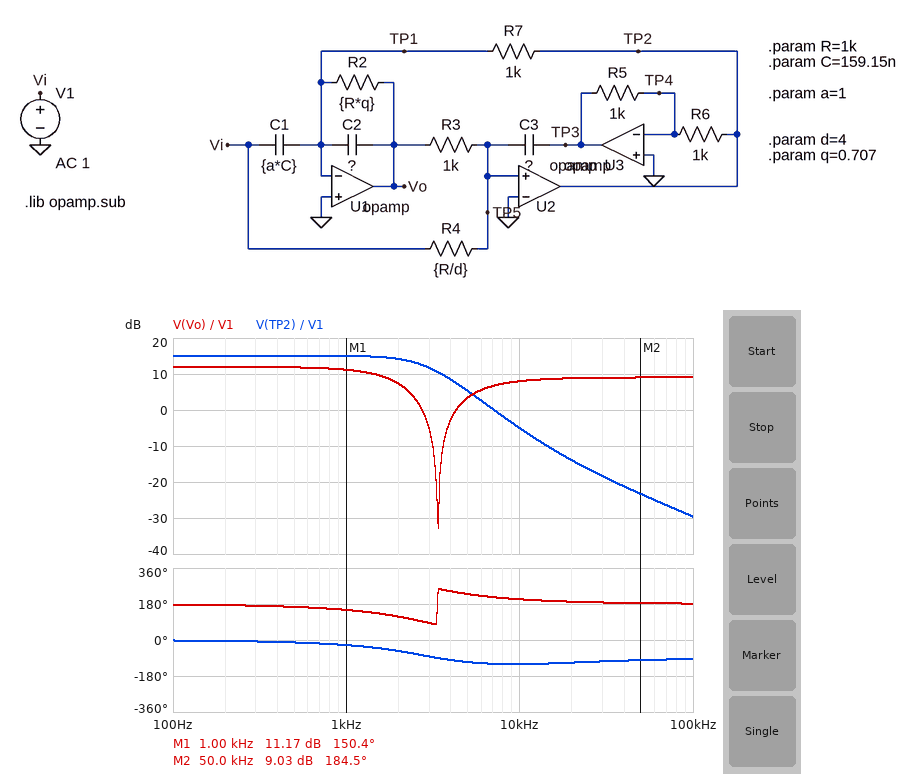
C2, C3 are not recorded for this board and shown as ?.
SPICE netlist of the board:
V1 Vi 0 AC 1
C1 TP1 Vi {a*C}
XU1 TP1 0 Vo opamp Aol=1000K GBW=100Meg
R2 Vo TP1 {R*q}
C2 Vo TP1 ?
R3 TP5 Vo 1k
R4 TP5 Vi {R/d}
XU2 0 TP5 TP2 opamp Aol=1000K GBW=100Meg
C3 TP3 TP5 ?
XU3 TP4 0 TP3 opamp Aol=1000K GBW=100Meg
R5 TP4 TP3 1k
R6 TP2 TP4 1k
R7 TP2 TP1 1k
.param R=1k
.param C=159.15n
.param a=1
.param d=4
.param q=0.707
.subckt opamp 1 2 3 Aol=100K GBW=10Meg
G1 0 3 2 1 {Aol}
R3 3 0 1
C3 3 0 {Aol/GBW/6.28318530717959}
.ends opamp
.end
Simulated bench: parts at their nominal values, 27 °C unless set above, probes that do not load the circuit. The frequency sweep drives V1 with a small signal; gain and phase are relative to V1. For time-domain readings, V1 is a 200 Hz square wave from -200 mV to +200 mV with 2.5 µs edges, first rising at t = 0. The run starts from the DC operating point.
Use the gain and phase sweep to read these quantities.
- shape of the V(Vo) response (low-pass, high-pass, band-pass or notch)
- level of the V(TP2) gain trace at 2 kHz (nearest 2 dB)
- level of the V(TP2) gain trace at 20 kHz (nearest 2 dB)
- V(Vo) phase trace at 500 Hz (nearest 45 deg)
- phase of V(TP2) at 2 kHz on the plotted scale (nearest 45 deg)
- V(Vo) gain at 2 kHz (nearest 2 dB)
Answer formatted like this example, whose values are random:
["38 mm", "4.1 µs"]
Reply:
["notch", "14 dB", "-14 dB", "180 deg", "-45 deg", "8 dB"]
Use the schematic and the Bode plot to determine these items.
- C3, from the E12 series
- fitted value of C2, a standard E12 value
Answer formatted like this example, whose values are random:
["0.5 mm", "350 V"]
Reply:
["56 nF", "56 nF"]
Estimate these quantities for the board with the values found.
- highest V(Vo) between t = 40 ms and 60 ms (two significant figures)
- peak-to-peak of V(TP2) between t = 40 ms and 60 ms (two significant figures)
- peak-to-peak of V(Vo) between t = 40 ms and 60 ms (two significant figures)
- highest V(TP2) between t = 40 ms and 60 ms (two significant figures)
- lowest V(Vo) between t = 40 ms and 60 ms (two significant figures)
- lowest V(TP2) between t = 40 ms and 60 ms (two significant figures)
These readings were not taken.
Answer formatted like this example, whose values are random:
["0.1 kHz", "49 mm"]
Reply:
["850 mV", "2.5 V", "1.7 V", "1.2 V", "-850 mV", "-1.2 V"]
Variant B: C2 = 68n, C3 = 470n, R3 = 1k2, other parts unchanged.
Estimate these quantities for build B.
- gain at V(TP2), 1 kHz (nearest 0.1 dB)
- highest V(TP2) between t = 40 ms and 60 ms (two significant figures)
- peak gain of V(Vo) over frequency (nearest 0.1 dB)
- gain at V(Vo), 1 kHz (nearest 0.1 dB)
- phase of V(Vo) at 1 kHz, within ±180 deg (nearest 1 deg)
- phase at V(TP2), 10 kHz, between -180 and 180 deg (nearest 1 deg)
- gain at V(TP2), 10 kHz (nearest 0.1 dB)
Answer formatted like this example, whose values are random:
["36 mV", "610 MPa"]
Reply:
["2.7 dB", "1.3 V", "13.6 dB", "-12.1 dB", "84 deg", "-104 deg", "-22.1 dB"]
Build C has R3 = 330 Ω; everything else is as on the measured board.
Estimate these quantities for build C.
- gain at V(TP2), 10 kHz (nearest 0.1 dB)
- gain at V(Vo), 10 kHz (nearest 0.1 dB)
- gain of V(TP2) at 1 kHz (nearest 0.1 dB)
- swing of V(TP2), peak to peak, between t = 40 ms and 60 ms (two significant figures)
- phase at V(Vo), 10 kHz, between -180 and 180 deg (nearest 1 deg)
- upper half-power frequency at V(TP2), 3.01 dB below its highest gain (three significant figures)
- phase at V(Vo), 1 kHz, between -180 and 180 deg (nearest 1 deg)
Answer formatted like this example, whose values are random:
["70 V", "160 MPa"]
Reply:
["4.2 dB", "9.4 dB", "6.0 dB", "1.5 V", "-152 deg", "6.83 kHz", "170 deg"]
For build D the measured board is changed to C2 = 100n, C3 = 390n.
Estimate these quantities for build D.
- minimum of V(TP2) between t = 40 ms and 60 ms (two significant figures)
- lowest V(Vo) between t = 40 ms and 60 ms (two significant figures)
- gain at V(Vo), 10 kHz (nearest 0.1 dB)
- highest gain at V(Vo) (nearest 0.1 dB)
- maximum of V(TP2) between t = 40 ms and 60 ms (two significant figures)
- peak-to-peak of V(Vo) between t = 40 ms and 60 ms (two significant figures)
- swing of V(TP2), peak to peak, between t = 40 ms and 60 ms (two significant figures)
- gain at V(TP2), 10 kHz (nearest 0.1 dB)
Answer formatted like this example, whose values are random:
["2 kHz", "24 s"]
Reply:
["-1.1 V", "-790 mV", "3.7 dB", "12.0 dB", "1.1 V", "1.6 V", "2.2 V", "-19.7 dB"]
